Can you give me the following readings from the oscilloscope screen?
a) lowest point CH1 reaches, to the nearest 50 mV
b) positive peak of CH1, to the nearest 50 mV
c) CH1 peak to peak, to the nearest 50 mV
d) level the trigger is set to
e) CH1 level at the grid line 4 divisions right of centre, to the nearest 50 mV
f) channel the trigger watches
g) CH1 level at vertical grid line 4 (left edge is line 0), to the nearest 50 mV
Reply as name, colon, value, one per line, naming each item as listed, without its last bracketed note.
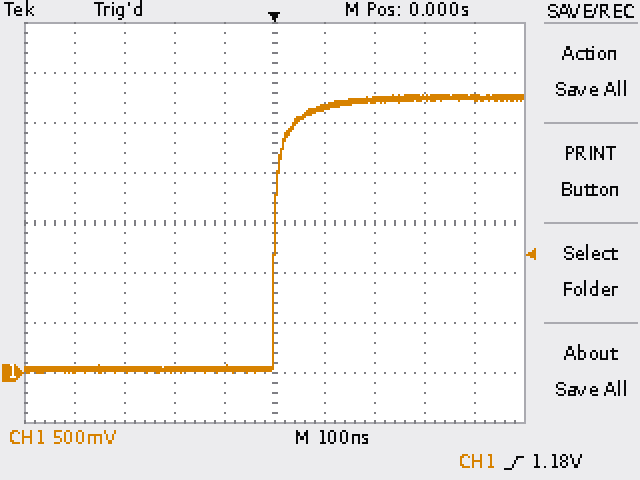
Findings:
lowest point CH1 reaches, to the nearest 50 mV: 0 mV
positive peak of CH1, to the nearest 50 mV: 2.80 V
CH1 peak to peak, to the nearest 50 mV: 2.80 V
level the trigger is set to: 1.18 V
CH1 level at the grid line 4 divisions right of centre, to the nearest 50 mV: 2.75 V
channel the trigger watches: CH1
CH1 level at vertical grid line 4 (left edge is line 0), to the nearest 50 mV: 50 mV
